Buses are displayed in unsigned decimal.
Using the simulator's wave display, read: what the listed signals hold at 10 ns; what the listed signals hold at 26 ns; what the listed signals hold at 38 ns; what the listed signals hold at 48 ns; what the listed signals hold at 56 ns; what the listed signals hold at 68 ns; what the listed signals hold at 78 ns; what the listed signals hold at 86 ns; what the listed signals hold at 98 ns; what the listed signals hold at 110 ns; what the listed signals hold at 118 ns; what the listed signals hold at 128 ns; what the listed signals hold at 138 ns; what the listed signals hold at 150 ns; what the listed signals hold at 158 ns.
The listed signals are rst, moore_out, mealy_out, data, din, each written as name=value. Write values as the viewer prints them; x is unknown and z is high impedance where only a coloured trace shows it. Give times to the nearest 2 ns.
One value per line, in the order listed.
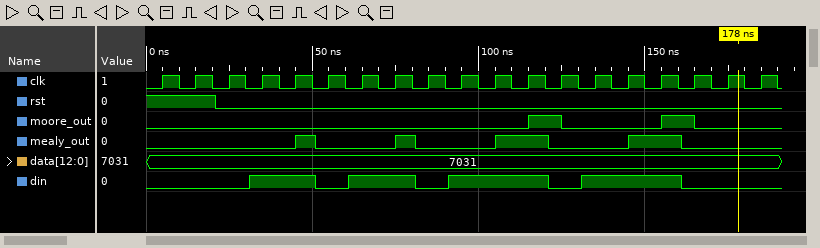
rst=1, moore_out=0, mealy_out=0, data=7031, din=0
rst=0, moore_out=0, mealy_out=0, data=7031, din=0
rst=0, moore_out=0, mealy_out=0, data=7031, din=1
rst=0, moore_out=0, mealy_out=1, data=7031, din=1
rst=0, moore_out=0, mealy_out=0, data=7031, din=0
rst=0, moore_out=0, mealy_out=0, data=7031, din=1
rst=0, moore_out=0, mealy_out=1, data=7031, din=1
rst=0, moore_out=0, mealy_out=0, data=7031, din=0
rst=0, moore_out=0, mealy_out=0, data=7031, din=1
rst=0, moore_out=0, mealy_out=1, data=7031, din=1
rst=0, moore_out=1, mealy_out=1, data=7031, din=1
rst=0, moore_out=0, mealy_out=0, data=7031, din=0
rst=0, moore_out=0, mealy_out=0, data=7031, din=1
rst=0, moore_out=0, mealy_out=1, data=7031, din=1
rst=0, moore_out=1, mealy_out=1, data=7031, din=1
